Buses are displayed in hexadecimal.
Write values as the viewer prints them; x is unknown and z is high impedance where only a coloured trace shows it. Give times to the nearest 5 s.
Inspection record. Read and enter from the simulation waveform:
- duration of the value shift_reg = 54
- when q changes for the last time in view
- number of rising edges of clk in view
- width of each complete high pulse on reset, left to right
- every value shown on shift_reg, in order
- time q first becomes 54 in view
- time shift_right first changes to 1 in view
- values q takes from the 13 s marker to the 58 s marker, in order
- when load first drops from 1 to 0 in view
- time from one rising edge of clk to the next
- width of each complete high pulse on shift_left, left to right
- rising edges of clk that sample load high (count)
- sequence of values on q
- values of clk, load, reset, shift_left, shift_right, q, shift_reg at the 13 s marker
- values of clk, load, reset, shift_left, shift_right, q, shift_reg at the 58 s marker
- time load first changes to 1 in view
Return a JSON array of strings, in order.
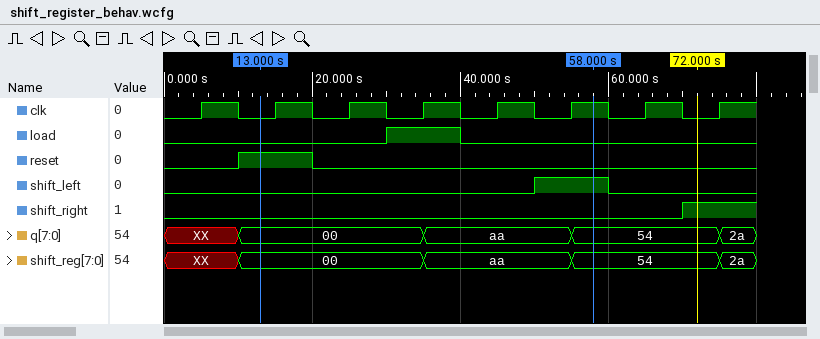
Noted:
["20 s", "75 s", "8", "10 s", "XX, 00, aa, 54, 2a", "55 s", "70 s", "00, aa, 54", "40 s", "10 s", "10 s", "1", "XX, 00, aa, 54, 2a", "clk=0, load=0, reset=1, shift_left=0, shift_right=0, q=00, shift_reg=00", "clk=1, load=0, reset=0, shift_left=1, shift_right=0, q=54, shift_reg=54", "30 s"]
